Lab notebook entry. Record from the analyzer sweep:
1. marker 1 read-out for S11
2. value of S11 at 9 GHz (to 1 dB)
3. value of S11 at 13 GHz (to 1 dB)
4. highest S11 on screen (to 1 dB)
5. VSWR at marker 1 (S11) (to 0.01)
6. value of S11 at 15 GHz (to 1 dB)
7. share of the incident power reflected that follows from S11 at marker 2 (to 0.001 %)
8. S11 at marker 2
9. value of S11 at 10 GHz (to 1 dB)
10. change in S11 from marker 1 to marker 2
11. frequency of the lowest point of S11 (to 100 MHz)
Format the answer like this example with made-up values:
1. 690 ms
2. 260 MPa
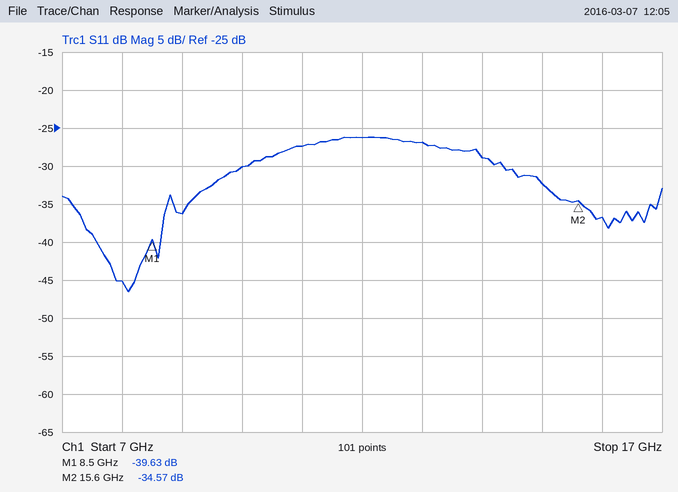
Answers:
1. -39.63 dB
2. -36 dB
3. -27 dB
4. -26 dB
5. 1.02
6. -32 dB
7. 0.035 %
8. -34.57 dB
9. -30 dB
10. 5.06 dB
11. 8.1 GHz
